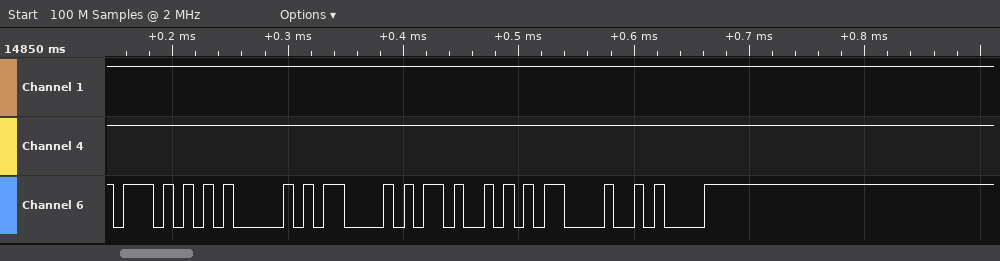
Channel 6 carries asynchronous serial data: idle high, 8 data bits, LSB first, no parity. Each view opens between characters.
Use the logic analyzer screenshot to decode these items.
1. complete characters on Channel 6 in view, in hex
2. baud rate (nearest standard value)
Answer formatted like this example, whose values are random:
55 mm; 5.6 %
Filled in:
57, 41, 43, 4B, 0D, 0A; 115200 baud
